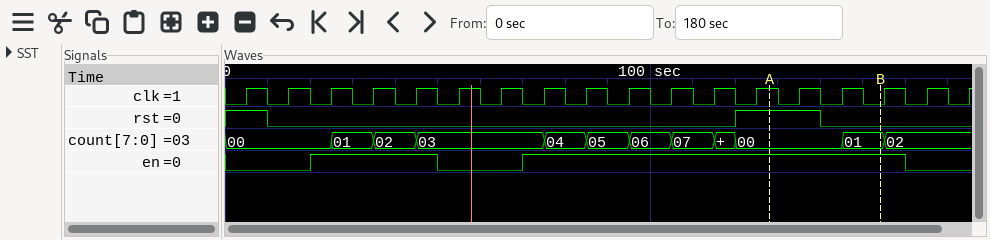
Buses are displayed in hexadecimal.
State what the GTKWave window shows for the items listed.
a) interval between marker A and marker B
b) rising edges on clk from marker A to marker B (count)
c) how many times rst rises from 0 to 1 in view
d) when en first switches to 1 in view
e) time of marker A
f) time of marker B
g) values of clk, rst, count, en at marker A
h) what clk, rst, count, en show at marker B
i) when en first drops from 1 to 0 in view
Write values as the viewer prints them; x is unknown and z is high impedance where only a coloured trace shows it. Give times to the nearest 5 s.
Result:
25 s
2
1
20 s
130 s
155 s
clk=1, rst=1, count=00, en=1
clk=0, rst=0, count=01, en=1
50 s
